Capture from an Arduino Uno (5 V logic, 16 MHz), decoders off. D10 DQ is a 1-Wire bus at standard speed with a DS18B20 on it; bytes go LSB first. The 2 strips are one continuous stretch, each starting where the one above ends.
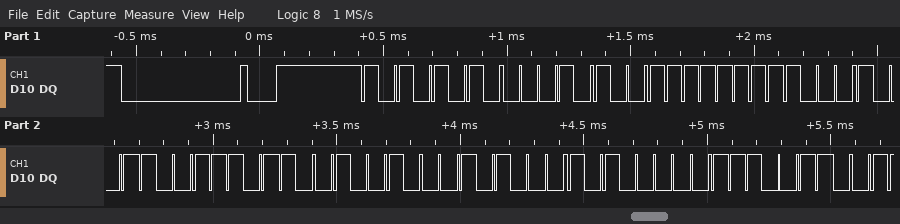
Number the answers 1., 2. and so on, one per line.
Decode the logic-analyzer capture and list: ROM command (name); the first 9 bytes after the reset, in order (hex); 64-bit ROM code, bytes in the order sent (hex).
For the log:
1. Match ROM
2. 55 28 FF 91 B9 49 14 05 67
3. 28 FF 91 B9 49 14 05 67
